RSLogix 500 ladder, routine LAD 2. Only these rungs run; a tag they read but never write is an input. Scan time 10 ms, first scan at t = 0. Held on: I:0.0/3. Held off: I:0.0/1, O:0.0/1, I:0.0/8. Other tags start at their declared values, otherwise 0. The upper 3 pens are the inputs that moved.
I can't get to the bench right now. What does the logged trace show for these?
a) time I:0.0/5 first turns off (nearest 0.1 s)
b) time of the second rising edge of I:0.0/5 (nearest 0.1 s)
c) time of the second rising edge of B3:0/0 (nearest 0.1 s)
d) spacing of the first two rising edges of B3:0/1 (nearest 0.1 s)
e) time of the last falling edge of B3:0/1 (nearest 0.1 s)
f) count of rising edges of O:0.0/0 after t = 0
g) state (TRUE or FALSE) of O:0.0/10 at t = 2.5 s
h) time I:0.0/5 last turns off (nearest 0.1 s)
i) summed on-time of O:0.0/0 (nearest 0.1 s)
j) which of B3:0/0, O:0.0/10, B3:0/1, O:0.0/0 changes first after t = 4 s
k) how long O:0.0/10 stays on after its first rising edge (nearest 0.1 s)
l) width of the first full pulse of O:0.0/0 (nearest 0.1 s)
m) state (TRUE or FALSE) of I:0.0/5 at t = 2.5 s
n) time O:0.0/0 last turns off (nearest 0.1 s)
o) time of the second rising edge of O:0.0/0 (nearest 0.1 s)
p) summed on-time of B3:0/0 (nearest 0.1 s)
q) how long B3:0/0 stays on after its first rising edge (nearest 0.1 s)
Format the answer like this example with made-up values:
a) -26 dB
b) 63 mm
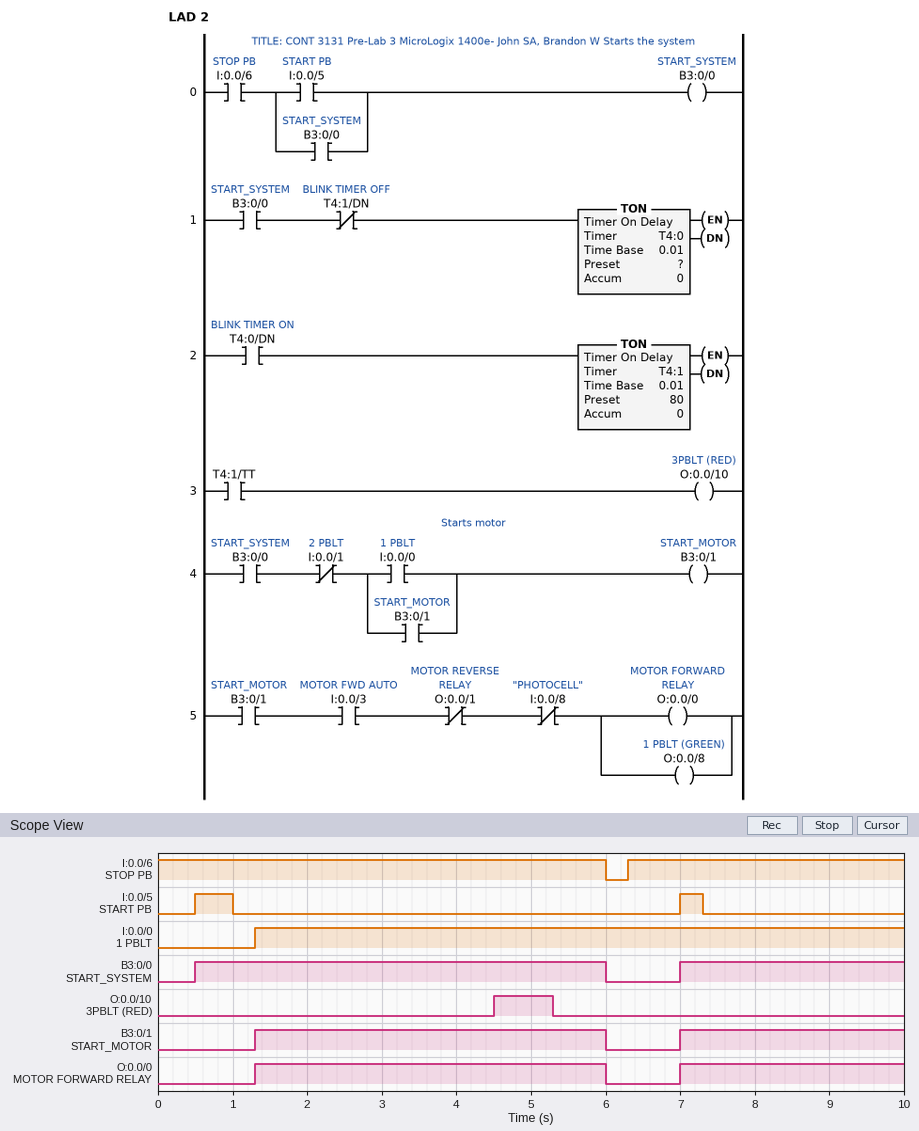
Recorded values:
a) 1.0 s
b) 7.0 s
c) 7.0 s
d) 5.7 s
e) 6.0 s
f) 2
g) FALSE
h) 7.3 s
i) 7.7 s
j) O:0.0/10
k) 0.8 s
l) 4.7 s
m) FALSE
n) 6.0 s
o) 7.0 s
p) 8.5 s
q) 5.5 s
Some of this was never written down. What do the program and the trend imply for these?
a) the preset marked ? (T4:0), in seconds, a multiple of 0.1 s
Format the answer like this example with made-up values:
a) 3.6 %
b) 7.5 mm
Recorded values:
a) 4.0 s
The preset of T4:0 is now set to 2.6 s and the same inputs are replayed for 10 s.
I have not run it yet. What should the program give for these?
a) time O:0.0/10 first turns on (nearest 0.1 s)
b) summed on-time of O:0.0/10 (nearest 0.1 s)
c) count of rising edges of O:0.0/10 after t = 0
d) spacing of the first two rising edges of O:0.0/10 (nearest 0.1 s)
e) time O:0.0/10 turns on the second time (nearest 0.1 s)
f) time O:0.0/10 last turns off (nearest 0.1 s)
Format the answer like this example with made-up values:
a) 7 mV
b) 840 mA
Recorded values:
a) 3.1 s
b) 1.2 s
c) 2
d) 6.5 s
e) 9.6 s
f) 3.9 s
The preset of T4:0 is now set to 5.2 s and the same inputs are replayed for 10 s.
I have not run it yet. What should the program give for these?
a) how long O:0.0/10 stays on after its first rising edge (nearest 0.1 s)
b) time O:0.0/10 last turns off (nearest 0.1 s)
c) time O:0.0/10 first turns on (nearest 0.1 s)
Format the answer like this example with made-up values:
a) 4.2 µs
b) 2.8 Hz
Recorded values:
a) 0.3 s
b) 6.0 s
c) 5.7 s
